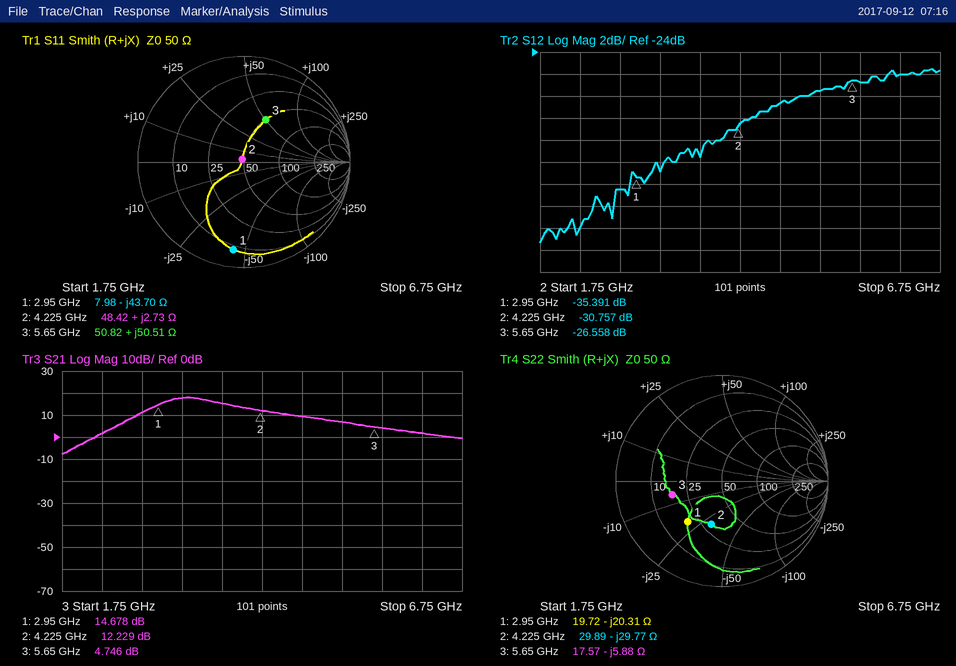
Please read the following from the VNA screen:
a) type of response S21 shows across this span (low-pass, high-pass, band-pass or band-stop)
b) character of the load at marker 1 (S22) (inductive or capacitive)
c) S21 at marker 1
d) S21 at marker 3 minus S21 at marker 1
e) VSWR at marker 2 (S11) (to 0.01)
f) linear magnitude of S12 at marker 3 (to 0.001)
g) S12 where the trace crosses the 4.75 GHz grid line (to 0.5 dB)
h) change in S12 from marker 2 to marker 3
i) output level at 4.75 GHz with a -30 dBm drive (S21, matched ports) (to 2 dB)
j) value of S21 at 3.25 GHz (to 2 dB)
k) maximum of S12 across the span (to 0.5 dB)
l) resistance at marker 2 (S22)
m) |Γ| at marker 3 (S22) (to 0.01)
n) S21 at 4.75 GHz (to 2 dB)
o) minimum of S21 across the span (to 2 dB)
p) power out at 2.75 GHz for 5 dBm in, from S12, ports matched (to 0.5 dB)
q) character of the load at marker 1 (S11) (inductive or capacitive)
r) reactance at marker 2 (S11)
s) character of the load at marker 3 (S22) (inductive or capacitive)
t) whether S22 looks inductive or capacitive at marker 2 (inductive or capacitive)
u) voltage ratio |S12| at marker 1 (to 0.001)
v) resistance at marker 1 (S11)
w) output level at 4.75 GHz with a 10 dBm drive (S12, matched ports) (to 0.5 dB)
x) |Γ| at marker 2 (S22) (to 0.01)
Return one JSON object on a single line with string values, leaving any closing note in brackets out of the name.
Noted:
{"type of response S21 shows across this span": "band-pass", "character of the load at marker 1 (S22)": "capacitive", "S21 at marker 1": "14.678 dB", "S21 at marker 3 minus S21 at marker 1": "-9.932 dB", "VSWR at marker 2 (S11)": "1.07", "linear magnitude of S12 at marker 3": "0.047", "S12 where the trace crosses the 4.75 GHz grid line": "-28.5 dB", "change in S12 from marker 2 to marker 3": "4.199 dB", "output level at 4.75 GHz with a -30 dBm drive (S21, matched ports)": "-20 dBm", "value of S21 at 3.25 GHz": "18 dB", "maximum of S12 across the span": "-25.5 dB", "resistance at marker 2": "29.89 Ω", "|Γ| at marker 3 (S22)": "0.49", "S21 at 4.75 GHz": "10 dB", "minimum of S21 across the span": "-8 dB", "power out at 2.75 GHz for 5 dBm in, from S12, ports matched": "-31.5 dBm", "character of the load at marker 1 (S11)": "capacitive", "reactance at marker 2": "+2.73 Ω", "character of the load at marker 3 (S22)": "capacitive", "whether S22 looks inductive or capacitive at marker 2": "capacitive", "voltage ratio |S12| at marker 1": "0.017", "resistance at marker 1": "7.98 Ω", "output level at 4.75 GHz with a 10 dBm drive (S12, matched ports)": "-18.5 dBm", "|Γ| at marker 2 (S22)": "0.42"}
